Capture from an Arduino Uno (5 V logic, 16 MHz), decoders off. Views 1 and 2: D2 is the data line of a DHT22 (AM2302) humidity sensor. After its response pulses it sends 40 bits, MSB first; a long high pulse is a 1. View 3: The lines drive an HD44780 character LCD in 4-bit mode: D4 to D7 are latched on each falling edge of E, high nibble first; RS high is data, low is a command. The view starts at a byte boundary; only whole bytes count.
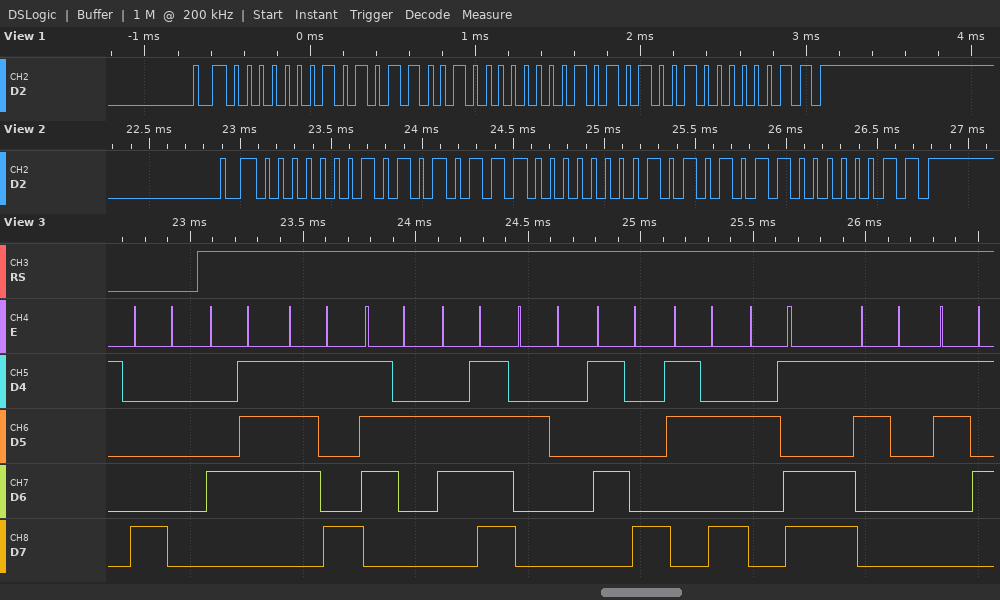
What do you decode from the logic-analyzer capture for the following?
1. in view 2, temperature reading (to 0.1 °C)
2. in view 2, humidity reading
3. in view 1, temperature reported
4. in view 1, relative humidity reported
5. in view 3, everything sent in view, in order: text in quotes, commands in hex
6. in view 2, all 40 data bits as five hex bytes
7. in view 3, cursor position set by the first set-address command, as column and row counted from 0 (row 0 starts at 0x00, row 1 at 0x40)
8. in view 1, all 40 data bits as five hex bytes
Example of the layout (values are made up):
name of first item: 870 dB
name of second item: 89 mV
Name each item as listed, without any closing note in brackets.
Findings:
in view 2, temperature reading: 17.1 °C
in view 2, humidity reading: 34.3 %
in view 1, temperature reported: 16.9 °C
in view 1, relative humidity reported: 34.5 %
in view 3, everything sent in view, in order: text in quotes, commands in hex: 0x80 "Gyro X:-15"
in view 2, all 40 data bits as five hex bytes: 01 57 00 AB 03
in view 3, cursor position set by the first set-address command, as column and row counted from 0: column 0, row 0
in view 1, all 40 data bits as five hex bytes: 01 59 00 A9 03
